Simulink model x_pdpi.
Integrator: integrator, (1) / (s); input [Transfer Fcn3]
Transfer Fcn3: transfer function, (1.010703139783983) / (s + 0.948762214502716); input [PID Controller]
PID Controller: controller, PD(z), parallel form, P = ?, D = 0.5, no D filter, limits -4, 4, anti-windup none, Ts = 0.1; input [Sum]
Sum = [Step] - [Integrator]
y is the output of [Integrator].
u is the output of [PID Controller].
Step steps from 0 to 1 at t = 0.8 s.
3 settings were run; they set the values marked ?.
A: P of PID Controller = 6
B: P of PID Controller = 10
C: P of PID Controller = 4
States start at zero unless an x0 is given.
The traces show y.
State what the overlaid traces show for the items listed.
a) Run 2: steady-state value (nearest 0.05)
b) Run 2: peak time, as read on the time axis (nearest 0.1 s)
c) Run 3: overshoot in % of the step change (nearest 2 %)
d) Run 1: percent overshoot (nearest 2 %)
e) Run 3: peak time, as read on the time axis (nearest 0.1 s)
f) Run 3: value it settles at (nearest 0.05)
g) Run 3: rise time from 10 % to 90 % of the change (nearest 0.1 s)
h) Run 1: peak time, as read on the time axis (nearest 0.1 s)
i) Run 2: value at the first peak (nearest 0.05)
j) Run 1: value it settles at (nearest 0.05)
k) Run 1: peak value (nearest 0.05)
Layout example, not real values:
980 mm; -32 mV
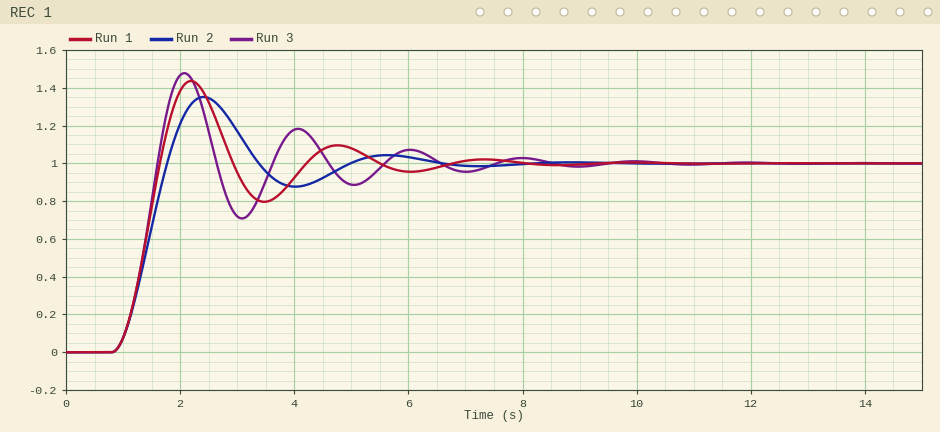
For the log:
1.00; 2.4 s; 48 %; 44 %; 2.1 s; 1.00; 0.5 s; 2.2 s; 1.35; 1.00; 1.45
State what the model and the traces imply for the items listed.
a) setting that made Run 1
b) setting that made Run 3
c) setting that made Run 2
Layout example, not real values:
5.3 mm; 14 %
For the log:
A; B; C
